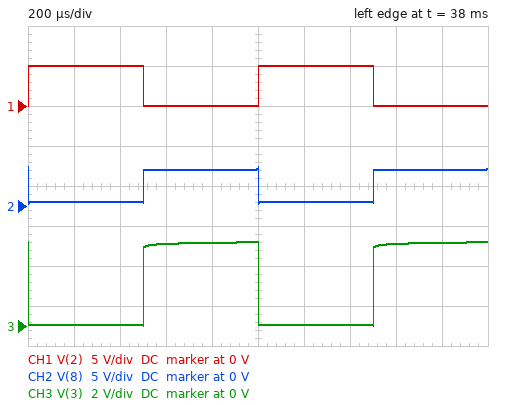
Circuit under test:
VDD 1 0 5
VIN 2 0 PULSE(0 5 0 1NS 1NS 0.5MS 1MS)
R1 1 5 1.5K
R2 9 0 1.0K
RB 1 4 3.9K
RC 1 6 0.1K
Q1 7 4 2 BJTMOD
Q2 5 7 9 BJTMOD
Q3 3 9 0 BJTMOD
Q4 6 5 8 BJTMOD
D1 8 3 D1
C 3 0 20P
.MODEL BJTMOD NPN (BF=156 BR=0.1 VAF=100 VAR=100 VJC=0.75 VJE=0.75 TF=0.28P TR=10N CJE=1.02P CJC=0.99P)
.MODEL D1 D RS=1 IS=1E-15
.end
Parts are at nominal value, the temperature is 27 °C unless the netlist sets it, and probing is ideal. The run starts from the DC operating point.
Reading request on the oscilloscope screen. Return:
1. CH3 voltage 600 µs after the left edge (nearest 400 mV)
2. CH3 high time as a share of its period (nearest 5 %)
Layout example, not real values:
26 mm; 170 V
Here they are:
4.0 V; 50 %
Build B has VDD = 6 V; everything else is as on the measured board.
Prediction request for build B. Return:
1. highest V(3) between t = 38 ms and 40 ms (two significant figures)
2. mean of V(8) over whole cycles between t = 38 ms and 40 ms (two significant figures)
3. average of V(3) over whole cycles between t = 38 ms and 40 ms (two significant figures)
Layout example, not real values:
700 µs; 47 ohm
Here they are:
5.2 V; 3.0 V; 2.6 V
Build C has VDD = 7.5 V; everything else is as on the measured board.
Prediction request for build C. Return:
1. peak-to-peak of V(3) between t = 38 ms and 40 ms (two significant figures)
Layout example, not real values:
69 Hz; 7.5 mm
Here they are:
6.7 V
